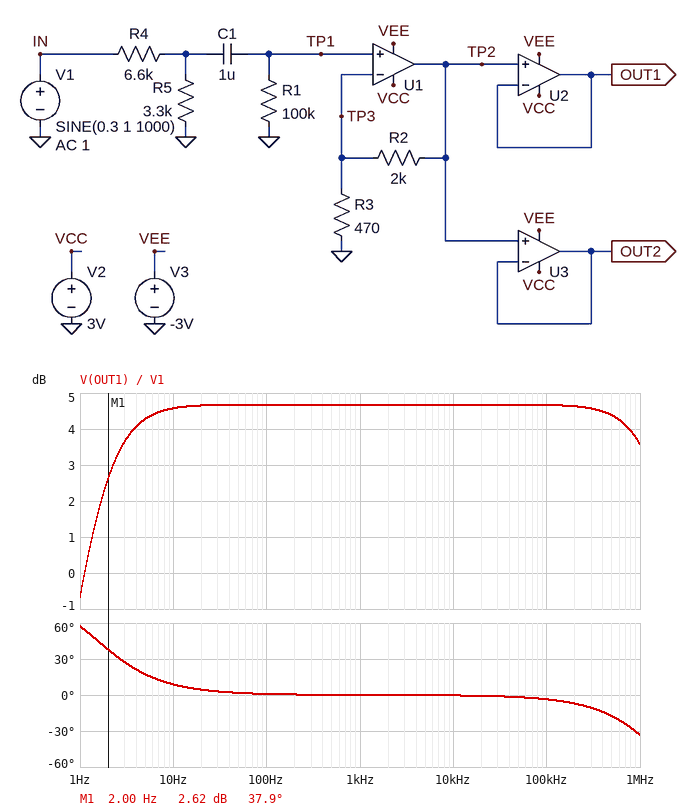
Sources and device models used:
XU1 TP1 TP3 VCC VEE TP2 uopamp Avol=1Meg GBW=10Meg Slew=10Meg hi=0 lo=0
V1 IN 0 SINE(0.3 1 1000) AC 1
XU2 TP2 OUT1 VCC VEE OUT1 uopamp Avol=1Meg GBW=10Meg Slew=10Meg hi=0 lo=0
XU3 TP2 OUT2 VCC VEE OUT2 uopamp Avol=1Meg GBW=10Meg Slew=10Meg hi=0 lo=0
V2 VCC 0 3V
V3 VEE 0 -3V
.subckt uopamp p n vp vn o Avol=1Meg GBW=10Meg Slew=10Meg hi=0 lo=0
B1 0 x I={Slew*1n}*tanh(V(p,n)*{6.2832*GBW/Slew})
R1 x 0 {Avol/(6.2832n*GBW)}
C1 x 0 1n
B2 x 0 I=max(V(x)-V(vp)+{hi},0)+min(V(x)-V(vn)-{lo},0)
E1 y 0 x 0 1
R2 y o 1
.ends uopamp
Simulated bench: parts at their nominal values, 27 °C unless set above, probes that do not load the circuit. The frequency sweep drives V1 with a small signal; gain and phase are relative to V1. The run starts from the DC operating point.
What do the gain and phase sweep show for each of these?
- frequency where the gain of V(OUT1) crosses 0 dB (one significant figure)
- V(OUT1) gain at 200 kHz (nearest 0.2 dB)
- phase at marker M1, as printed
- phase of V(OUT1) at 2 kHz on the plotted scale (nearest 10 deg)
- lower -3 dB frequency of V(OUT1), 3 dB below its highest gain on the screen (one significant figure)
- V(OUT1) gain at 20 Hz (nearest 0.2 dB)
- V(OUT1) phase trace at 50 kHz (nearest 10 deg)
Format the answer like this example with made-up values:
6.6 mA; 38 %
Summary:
1 Hz; 4.6 dB; 37.9 deg; 0 deg; 2 Hz; 4.6 dB; 0 deg
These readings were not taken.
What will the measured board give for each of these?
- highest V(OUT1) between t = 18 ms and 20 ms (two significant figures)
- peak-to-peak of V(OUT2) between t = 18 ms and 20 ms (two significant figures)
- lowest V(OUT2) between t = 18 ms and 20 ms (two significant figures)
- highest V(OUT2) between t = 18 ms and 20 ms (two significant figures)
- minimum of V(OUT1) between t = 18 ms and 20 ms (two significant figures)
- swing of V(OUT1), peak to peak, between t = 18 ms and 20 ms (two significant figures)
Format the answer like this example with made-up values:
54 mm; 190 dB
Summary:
1.7 V; 3.4 V; -1.7 V; 1.7 V; -1.7 V; 3.4 V
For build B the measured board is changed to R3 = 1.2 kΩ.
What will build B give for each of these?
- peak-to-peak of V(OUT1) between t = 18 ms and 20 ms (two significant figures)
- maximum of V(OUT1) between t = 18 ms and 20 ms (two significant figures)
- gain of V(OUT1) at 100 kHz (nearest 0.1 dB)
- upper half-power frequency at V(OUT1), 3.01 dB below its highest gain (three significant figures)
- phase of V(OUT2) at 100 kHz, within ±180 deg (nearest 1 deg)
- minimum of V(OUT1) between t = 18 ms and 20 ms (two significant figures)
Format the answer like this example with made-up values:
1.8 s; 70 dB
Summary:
1.7 V; 870 mV; -1.2 dB; 3.35 MHz; -2 deg; -870 mV
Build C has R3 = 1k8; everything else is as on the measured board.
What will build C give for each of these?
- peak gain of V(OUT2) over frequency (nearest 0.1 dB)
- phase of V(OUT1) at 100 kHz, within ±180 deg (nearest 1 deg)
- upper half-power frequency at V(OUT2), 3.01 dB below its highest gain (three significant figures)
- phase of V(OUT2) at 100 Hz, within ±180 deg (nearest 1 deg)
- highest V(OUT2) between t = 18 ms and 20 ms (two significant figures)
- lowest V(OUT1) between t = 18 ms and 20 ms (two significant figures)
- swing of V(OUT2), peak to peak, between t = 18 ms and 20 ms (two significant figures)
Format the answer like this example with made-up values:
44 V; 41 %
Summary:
-3.2 dB; -2 deg; 4.02 MHz; 1 deg; 690 mV; -690 mV; 1.4 V
